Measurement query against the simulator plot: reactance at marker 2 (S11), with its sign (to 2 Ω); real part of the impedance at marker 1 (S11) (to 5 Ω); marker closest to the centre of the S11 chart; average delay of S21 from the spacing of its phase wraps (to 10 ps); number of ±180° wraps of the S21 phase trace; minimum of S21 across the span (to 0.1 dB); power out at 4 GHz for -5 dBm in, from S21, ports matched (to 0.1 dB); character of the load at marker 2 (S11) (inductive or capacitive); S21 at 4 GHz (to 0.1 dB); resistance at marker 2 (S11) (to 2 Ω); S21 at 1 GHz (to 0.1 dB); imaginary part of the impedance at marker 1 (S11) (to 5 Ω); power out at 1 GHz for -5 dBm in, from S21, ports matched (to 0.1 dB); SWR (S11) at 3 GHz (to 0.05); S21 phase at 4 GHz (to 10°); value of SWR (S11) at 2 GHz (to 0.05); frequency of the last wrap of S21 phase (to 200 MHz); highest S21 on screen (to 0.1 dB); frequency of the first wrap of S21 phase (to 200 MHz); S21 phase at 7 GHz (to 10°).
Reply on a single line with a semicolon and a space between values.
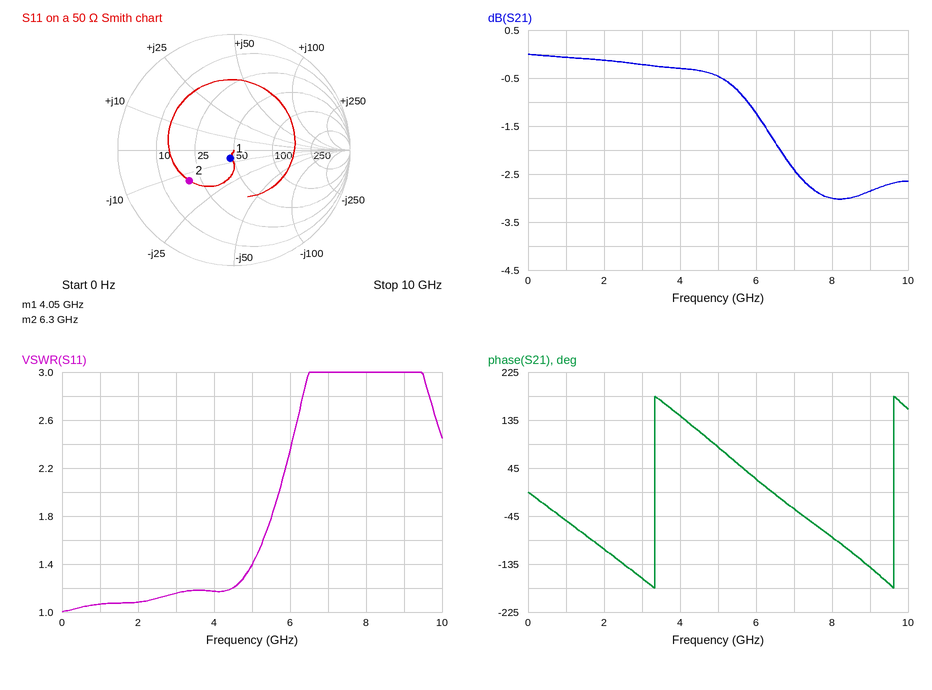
-14 Ω; 45 Ω; marker 1; 160 ps; 2; -3.0 dB; -5.3 dBm; capacitive; -0.3 dB; 20 Ω; -0.1 dB; -5 Ω; -5.1 dBm; 1.15; 140°; 1.10; 9.6 GHz; 0.0 dB; 3.4 GHz; -30°
